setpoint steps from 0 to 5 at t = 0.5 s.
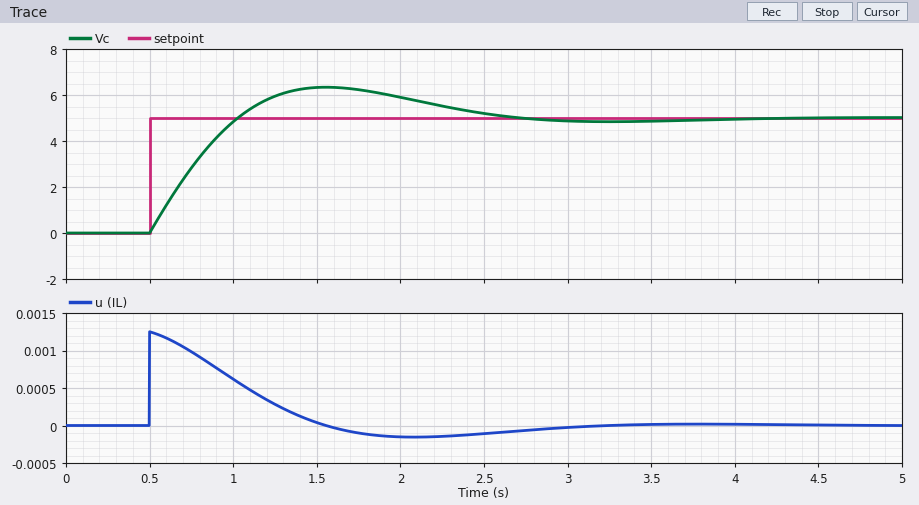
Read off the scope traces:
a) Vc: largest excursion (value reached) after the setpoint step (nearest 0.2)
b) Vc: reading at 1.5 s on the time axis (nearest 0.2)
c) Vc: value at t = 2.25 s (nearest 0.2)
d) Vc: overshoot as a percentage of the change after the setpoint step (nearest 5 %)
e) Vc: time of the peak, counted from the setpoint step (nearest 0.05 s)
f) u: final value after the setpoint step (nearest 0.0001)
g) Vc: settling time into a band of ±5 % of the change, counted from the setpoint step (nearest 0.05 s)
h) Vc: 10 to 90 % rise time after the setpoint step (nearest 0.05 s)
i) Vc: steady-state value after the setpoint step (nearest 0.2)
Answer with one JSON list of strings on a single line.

["6.4", "6.4", "5.6", "25 %", "1.05 s", "0.0000", "1.95 s", "0.40 s", "5.0"]
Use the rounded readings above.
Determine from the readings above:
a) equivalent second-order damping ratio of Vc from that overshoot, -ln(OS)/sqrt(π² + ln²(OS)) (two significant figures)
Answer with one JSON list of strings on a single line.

["0.40"]
